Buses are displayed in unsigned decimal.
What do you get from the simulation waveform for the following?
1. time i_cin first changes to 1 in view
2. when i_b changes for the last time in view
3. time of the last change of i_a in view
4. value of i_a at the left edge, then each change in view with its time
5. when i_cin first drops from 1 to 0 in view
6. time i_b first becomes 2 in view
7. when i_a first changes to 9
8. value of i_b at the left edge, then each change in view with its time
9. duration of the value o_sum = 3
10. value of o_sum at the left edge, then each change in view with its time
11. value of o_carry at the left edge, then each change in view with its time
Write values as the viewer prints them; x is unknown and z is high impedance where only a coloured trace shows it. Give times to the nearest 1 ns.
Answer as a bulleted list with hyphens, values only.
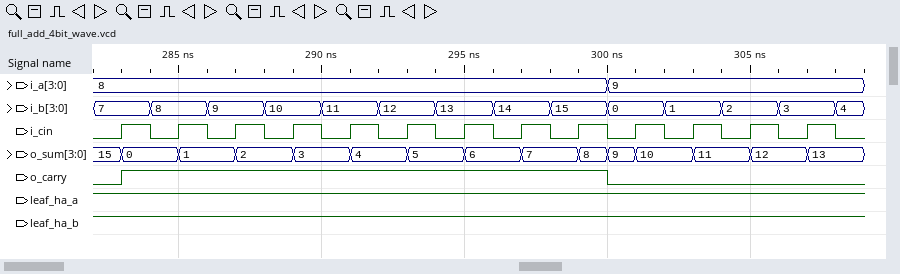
- 283 ns
- 308 ns
- 300 ns
- 8, 9 at 300 ns
- 284 ns
- 304 ns
- 300 ns
- 7, 8 at 284 ns, 9 at 286 ns, 10 at 288 ns, 11 at 290 ns, 12 at 292 ns, 13 at 294 ns, 14 at 296 ns, 15 at 298 ns, 0 at 300 ns, 1 at 302 ns, 2 at 304 ns, 3 at 306 ns, 4 at 308 ns
- 2 ns
- 15, 0 at 283 ns, 1 at 285 ns, 2 at 287 ns, 3 at 289 ns, 4 at 291 ns, 5 at 293 ns, 6 at 295 ns, 7 at 297 ns, 8 at 299 ns, 9 at 300 ns, 10 at 301 ns, 11 at 303 ns, 12 at 305 ns, 13 at 307 ns
- 0, 1 at 283 ns, 0 at 300 ns
